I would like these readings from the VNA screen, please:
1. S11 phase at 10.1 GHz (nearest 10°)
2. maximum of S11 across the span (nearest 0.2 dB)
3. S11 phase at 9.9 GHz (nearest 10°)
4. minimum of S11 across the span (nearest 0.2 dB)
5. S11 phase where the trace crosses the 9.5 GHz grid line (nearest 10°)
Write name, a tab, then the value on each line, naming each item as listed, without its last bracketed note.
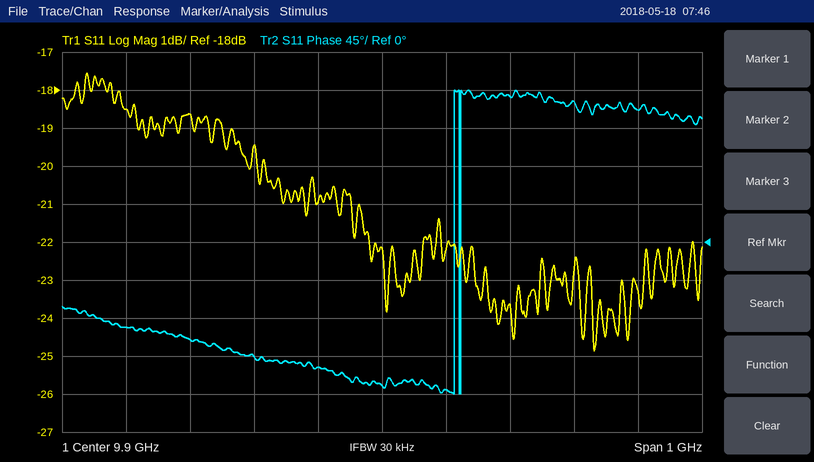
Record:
S11 phase at 10.1 GHz	170°
maximum of S11 across the span	-17.6 dB
S11 phase at 9.9 GHz	-170°
minimum of S11 across the span	-24.8 dB
S11 phase where the trace crosses the 9.5 GHz grid line	-100°
